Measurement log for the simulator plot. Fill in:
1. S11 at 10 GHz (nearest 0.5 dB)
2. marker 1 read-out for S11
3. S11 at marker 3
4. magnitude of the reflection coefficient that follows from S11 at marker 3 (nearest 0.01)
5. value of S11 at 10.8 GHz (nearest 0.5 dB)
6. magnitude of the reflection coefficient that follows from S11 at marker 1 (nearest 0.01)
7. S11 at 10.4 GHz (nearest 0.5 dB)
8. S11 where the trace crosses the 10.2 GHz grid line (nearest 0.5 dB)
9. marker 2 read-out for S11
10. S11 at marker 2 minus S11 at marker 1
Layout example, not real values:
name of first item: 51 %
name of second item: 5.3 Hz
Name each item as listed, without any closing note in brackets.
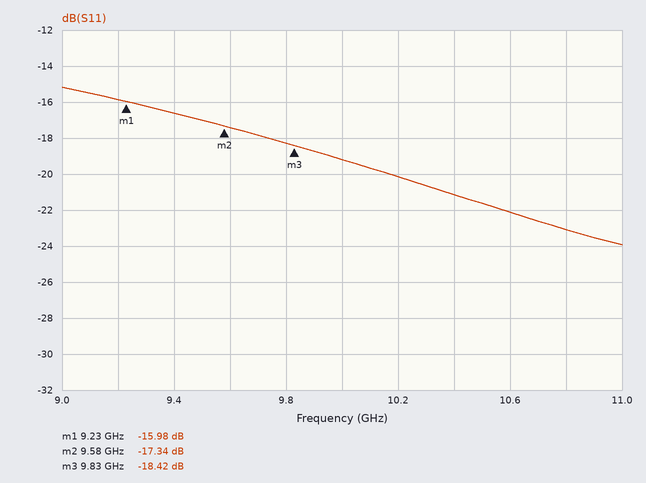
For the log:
S11 at 10 GHz: -19.0 dB
marker 1 read-out for S11: -15.98 dB
S11 at marker 3: -18.42 dB
magnitude of the reflection coefficient that follows from S11 at marker 3: 0.12
value of S11 at 10.8 GHz: -23.0 dB
magnitude of the reflection coefficient that follows from S11 at marker 1: 0.16
S11 at 10.4 GHz: -21.0 dB
S11 where the trace crosses the 10.2 GHz grid line: -20.0 dB
marker 2 read-out for S11: -17.34 dB
S11 at marker 2 minus S11 at marker 1: -1.36 dB
